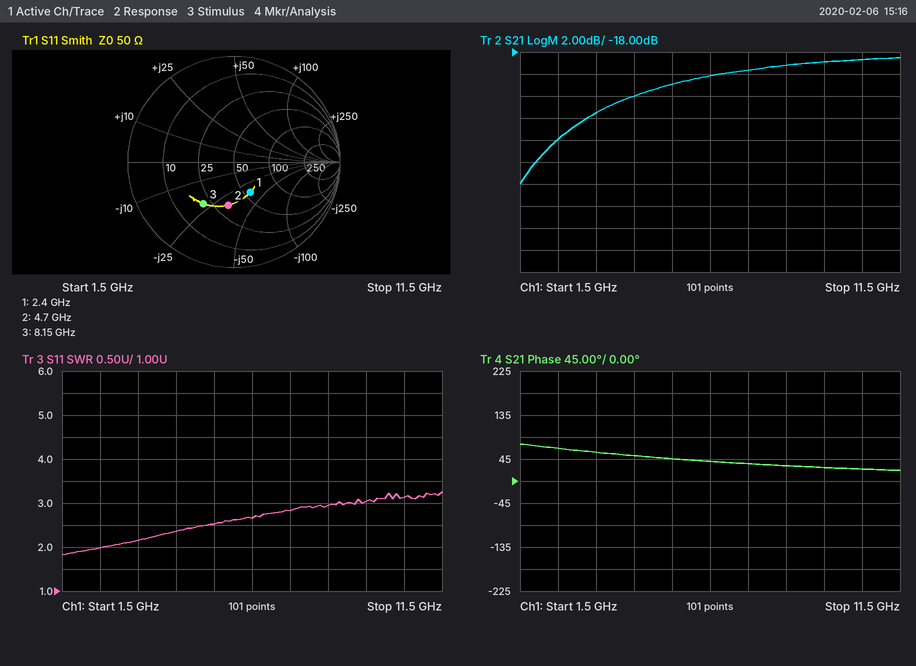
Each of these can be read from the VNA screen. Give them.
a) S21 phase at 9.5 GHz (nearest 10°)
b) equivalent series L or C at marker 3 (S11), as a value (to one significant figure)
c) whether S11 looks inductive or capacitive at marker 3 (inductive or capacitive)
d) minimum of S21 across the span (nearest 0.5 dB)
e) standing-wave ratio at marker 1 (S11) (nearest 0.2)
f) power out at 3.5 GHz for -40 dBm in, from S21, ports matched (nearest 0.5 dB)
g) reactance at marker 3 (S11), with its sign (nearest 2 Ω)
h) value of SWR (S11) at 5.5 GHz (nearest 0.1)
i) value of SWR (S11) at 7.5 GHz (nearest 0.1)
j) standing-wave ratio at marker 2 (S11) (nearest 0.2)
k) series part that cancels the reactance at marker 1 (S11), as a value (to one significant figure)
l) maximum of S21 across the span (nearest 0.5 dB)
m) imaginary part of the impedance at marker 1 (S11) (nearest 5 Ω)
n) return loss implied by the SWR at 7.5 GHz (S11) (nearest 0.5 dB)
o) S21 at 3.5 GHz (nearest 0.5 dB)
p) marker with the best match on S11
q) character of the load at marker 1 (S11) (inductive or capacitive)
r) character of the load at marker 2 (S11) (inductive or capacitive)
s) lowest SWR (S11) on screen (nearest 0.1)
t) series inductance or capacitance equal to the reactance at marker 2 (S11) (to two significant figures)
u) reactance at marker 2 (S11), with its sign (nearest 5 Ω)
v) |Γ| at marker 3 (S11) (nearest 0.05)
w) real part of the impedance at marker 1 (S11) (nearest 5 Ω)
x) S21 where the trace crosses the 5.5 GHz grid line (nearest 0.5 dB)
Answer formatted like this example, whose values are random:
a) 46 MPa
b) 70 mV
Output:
a) 30°
b) 900 fF
c) capacitive
d) -30.0 dB
e) 2.0
f) -63.5 dBm
g) -22 Ω
h) 2.5
i) 2.8
j) 2.4
k) 2 nH
l) -18.5 dB
m) -35 Ω
n) 6.5 dB
o) -23.5 dB
p) marker 1
q) capacitive
r) capacitive
s) 1.8
t) 1.1 pF
u) -30 Ω
v) 0.50
w) 55 Ω
x) -21.0 dB
